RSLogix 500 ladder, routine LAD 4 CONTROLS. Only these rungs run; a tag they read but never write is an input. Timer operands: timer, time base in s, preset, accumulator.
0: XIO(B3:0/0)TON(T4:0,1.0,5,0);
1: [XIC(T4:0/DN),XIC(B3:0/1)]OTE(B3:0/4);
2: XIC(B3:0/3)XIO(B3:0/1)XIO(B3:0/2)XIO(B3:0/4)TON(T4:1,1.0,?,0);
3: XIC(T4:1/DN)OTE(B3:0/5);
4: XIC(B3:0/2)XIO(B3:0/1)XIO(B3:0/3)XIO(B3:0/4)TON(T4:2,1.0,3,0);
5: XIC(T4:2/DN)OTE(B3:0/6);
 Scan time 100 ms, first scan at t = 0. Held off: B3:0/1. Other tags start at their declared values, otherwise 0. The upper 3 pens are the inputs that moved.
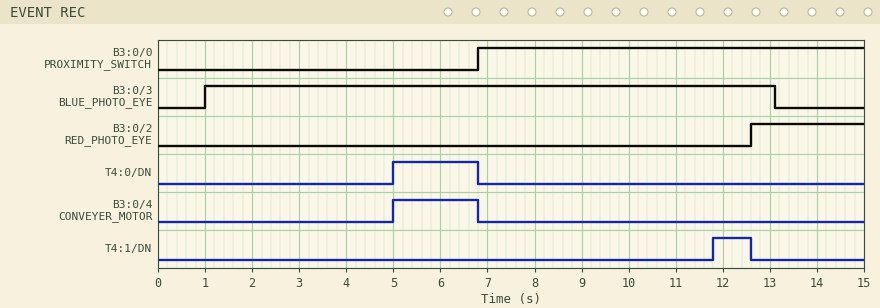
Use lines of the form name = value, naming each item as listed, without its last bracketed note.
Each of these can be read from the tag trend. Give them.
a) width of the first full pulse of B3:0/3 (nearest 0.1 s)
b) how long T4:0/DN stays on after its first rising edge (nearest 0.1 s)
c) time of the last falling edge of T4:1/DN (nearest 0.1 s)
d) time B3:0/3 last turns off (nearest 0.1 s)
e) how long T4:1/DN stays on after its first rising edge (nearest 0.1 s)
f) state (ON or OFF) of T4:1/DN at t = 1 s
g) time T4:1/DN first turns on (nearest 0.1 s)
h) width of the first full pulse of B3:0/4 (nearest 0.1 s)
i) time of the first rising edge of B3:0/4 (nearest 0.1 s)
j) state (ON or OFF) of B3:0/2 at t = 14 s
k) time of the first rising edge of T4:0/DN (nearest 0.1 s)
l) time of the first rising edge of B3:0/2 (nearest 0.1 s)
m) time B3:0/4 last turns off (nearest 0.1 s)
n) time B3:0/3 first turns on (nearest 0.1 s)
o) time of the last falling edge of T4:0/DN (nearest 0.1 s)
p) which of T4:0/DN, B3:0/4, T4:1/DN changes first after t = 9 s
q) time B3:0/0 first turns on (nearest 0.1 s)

width of the first full pulse of B3:0/3 = 12.1 s
how long T4:0/DN stays on after its first rising edge = 1.8 s
time of the last falling edge of T4:1/DN = 12.6 s
time B3:0/3 last turns off = 13.1 s
how long T4:1/DN stays on after its first rising edge = 0.8 s
state (ON or OFF) of T4:1/DN at t = 1 s = OFF
time T4:1/DN first turns on = 11.8 s
width of the first full pulse of B3:0/4 = 1.8 s
time of the first rising edge of B3:0/4 = 5.0 s
state (ON or OFF) of B3:0/2 at t = 14 s = ON
time of the first rising edge of T4:0/DN = 5.0 s
time of the first rising edge of B3:0/2 = 12.6 s
time B3:0/4 last turns off = 6.8 s
time B3:0/3 first turns on = 1.0 s
time of the last falling edge of T4:0/DN = 6.8 s
which of T4:0/DN, B3:0/4, T4:1/DN changes first after t = 9 s = T4:1/DN
time B3:0/0 first turns on = 6.8 s
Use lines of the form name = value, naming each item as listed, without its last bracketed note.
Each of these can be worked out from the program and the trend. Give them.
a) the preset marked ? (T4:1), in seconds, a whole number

the preset marked ? (T4:1), in seconds, a whole number = 5 s
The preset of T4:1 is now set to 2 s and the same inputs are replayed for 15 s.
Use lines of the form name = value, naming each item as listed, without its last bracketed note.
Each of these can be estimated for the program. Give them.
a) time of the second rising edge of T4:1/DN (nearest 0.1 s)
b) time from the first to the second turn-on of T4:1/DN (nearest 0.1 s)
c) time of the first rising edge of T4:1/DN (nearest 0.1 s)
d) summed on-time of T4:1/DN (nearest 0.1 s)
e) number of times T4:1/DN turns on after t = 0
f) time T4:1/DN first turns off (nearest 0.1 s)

time of the second rising edge of T4:1/DN = 8.8 s
time from the first to the second turn-on of T4:1/DN = 5.8 s
time of the first rising edge of T4:1/DN = 3.0 s
summed on-time of T4:1/DN = 5.8 s
number of times T4:1/DN turns on after t = 0 = 2
time T4:1/DN first turns off = 5.0 s
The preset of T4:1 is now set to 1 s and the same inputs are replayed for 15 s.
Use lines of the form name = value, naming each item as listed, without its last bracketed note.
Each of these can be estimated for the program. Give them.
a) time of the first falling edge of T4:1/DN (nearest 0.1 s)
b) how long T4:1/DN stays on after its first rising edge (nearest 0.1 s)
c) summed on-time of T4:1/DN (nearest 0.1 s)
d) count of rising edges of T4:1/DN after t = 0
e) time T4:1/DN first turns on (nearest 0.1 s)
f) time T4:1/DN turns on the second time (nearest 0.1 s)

time of the first falling edge of T4:1/DN = 5.0 s
how long T4:1/DN stays on after its first rising edge = 3.0 s
summed on-time of T4:1/DN = 7.8 s
count of rising edges of T4:1/DN after t = 0 = 2
time T4:1/DN first turns on = 2.0 s
time T4:1/DN turns on the second time = 7.8 s
